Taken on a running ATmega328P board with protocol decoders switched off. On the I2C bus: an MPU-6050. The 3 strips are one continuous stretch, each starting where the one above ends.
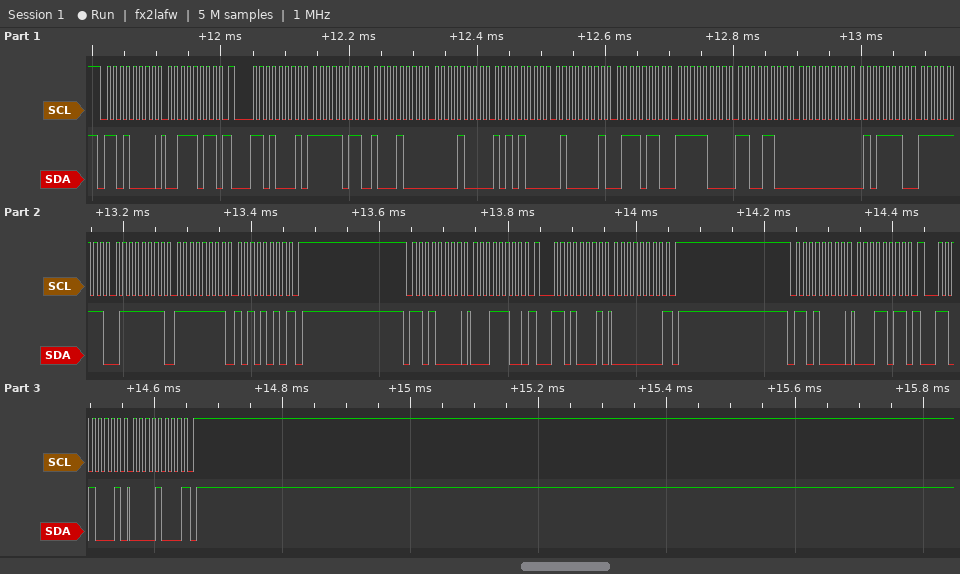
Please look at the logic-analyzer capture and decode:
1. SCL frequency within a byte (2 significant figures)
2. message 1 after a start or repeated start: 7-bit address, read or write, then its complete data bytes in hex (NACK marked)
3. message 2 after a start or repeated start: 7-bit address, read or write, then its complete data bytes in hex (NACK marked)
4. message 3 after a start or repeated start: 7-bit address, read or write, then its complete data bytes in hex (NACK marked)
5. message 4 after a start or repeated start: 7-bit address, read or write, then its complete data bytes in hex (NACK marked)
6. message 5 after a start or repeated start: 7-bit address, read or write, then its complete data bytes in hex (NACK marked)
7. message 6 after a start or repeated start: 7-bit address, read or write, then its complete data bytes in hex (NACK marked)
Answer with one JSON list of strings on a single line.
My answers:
["100 kHz", "0x68 write: 3B", "0x68 read: FB 88 08 A8 41 76 F8 CC 00 5E FF 7F FF AA NACK", "0x68 write: 1C", "0x68 read: 00 NACK", "0x68 write: 1B", "0x68 read: 08 NACK"]
